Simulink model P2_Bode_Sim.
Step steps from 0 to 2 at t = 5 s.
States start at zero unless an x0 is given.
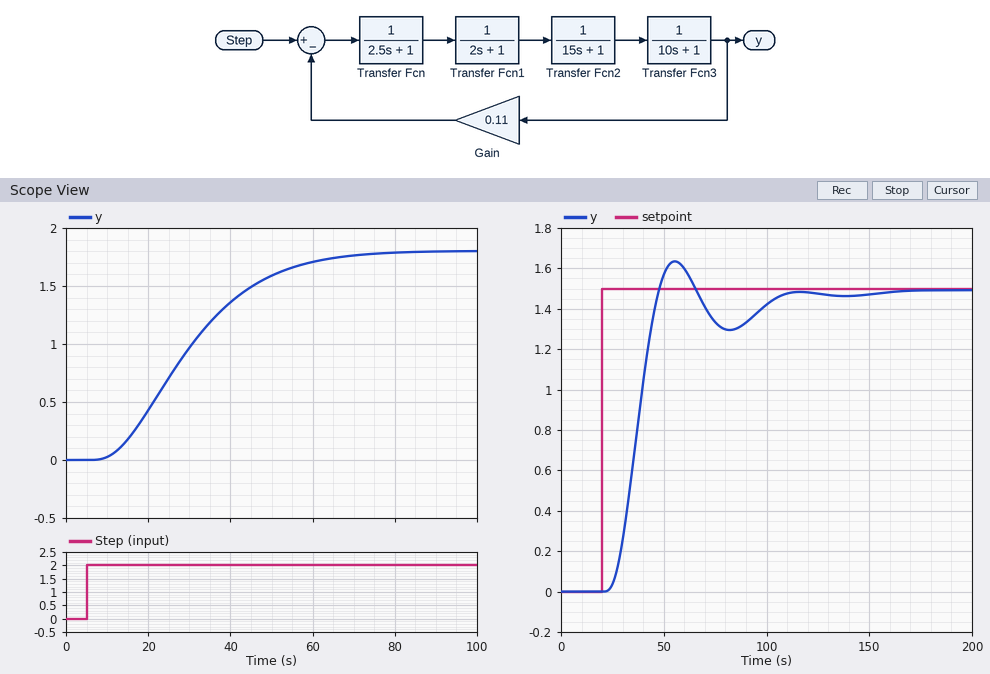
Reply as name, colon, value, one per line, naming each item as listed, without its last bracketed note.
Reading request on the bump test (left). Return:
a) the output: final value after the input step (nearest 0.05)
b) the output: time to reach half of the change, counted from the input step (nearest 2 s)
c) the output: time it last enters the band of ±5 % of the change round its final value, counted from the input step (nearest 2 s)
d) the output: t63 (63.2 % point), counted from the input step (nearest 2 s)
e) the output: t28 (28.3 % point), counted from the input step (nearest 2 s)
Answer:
the output: final value after the input step: 1.80
the output: time to reach half of the change, counted from the input step: 24 s
the output: time it last enters the band of ±5 % of the change round its final value, counted from the input step: 56 s
the output: t63 (63.2 % point), counted from the input step: 28 s
the output: t28 (28.3 % point), counted from the input step: 16 s
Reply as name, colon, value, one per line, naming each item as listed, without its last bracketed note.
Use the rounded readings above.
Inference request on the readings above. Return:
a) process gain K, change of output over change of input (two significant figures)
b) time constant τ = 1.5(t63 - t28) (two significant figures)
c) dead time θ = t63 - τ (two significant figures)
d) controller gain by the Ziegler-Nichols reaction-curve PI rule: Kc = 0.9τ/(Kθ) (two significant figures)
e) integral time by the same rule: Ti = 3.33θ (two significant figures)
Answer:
process gain K, change of output over change of input: 0.90
time constant τ = 1.5(t63 - t28): 18 s
dead time θ = t63 - τ: 10 s
controller gain by the Ziegler-Nichols reaction-curve PI rule: Kc = 0.9τ/(Kθ): 1.8
integral time by the same rule: Ti = 3.33θ: 33 s
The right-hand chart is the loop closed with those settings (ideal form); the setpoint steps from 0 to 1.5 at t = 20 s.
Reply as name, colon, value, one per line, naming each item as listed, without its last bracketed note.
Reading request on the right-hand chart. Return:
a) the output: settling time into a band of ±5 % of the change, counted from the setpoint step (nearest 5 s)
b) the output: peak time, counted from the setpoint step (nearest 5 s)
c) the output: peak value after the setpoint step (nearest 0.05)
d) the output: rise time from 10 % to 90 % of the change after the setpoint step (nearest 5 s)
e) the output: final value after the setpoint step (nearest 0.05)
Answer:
the output: settling time into a band of ±5 % of the change, counted from the setpoint step: 80 s
the output: peak time, counted from the setpoint step: 35 s
the output: peak value after the setpoint step: 1.65
the output: rise time from 10 % to 90 % of the change after the setpoint step: 15 s
the output: final value after the setpoint step: 1.50
